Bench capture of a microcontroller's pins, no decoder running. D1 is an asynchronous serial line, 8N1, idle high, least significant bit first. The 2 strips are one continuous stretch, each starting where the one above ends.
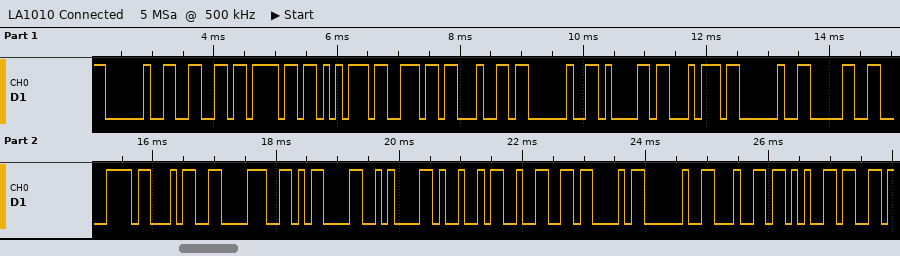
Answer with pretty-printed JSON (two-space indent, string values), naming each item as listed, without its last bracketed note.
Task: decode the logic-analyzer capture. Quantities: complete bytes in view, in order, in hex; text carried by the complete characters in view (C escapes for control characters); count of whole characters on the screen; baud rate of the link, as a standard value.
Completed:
{
  "complete bytes in view, in order, in hex": "20 66 6F 75 6E 64 20 61 74 20 30 78 34 38 0D 0A 49 32 43 20 64 65",
  "text carried by the complete characters in view": "\" found at 0x48\\r\\nI2C de\"",
  "count of whole characters on the screen": "22",
  "baud rate of the link, as a standard value": "9600 baud"
}
